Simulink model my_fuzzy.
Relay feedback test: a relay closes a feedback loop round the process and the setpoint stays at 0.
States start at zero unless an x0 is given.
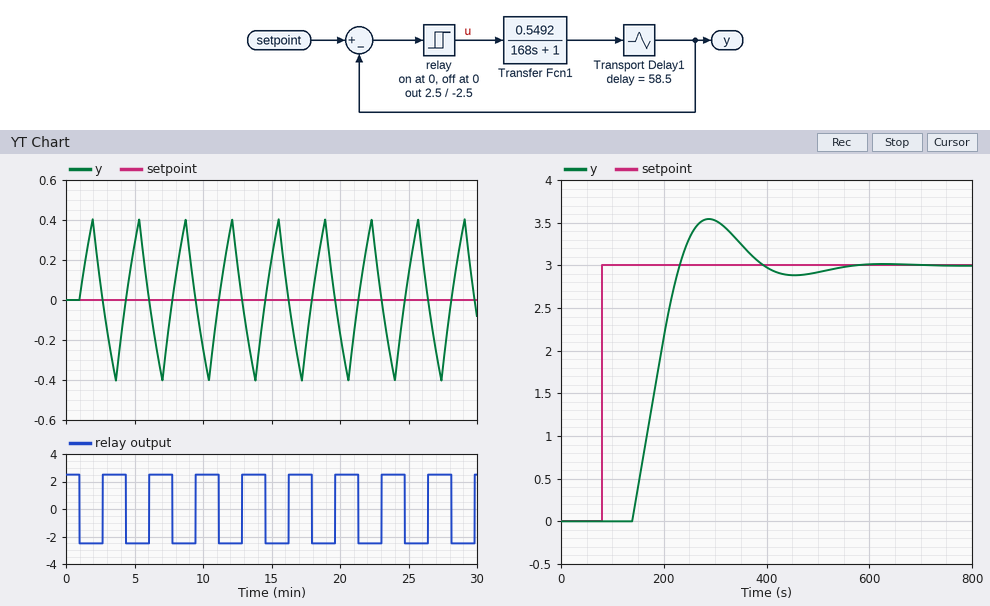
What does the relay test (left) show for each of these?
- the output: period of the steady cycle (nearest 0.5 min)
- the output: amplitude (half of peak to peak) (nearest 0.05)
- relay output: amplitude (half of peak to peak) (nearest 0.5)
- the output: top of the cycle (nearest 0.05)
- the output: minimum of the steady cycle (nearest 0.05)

3.5 min
0.40
2.5
0.40
-0.40
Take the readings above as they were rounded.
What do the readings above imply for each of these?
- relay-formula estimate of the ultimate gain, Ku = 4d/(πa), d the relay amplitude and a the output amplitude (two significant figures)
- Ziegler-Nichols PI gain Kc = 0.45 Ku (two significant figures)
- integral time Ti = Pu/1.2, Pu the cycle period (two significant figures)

8.0
3.6
2.9 min
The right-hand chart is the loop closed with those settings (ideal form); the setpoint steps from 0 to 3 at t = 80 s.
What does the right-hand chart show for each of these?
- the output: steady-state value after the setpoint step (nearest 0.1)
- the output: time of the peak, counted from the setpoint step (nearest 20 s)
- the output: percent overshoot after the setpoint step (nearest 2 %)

3.0
200 s
18 %
